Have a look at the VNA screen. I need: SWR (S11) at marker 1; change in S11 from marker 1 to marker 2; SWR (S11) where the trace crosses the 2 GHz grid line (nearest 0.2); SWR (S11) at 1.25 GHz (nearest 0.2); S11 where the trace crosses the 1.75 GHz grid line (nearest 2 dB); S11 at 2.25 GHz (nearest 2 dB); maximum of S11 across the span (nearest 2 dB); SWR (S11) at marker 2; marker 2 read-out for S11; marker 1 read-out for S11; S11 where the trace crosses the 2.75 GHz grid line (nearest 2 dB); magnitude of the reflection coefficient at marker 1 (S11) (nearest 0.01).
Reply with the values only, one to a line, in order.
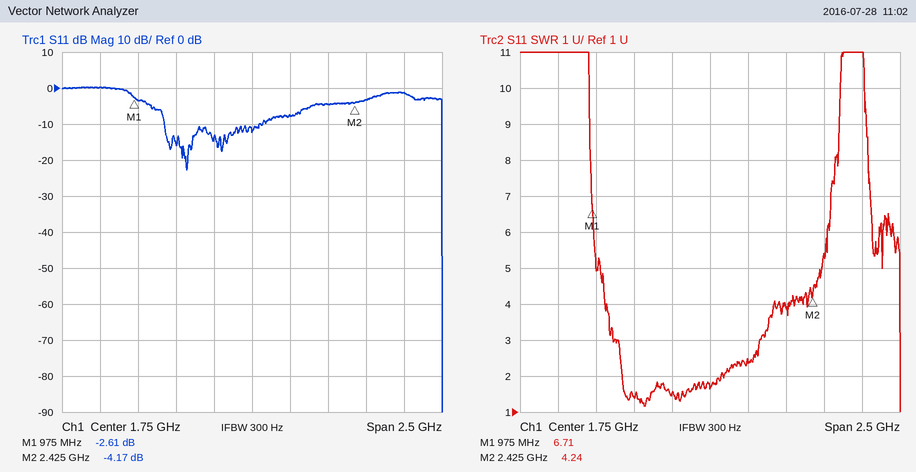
6.71
-1.56 dB
2.4
1.4
-12 dB
-4 dB
0 dB
4.24
-4.17 dB
-2.61 dB
-2 dB
0.74
